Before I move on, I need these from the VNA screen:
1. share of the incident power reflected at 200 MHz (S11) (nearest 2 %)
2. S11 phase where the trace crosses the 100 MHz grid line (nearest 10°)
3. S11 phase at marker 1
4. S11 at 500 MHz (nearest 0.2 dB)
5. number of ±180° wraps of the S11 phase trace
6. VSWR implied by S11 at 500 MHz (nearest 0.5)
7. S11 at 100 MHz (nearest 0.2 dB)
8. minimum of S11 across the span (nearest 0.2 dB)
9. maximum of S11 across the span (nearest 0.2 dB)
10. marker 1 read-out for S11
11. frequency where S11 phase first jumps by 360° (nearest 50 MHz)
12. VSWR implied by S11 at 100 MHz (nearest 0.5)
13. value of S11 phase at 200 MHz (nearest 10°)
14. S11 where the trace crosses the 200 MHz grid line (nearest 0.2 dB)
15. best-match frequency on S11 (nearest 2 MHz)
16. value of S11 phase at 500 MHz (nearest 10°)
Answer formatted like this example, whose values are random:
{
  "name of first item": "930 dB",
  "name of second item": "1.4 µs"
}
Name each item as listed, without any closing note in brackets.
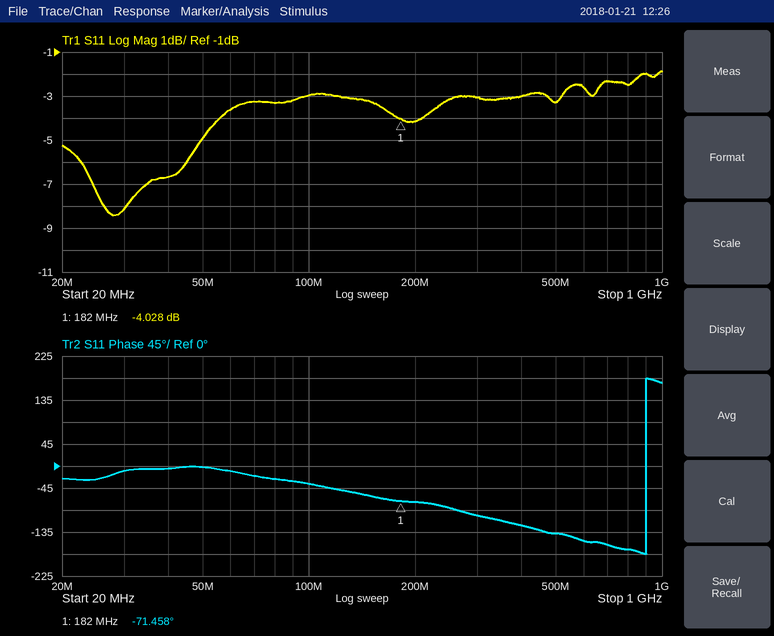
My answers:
{
  "share of the incident power reflected at 200 MHz (S11)": "38 %",
  "S11 phase where the trace crosses the 100 MHz grid line": "-40°",
  "S11 phase at marker 1": "-71.458°",
  "S11 at 500 MHz": "-3.2 dB",
  "number of ±180° wraps of the S11 phase trace": "1",
  "VSWR implied by S11 at 500 MHz": "5.5",
  "S11 at 100 MHz": "-3.0 dB",
  "minimum of S11 across the span": "-8.4 dB",
  "maximum of S11 across the span": "-1.8 dB",
  "marker 1 read-out for S11": "-4.028 dB",
  "frequency where S11 phase first jumps by 360°": "900 MHz",
  "VSWR implied by S11 at 100 MHz": "6.0",
  "value of S11 phase at 200 MHz": "-70°",
  "S11 where the trace crosses the 200 MHz grid line": "-4.2 dB",
  "best-match frequency on S11": "28 MHz",
  "value of S11 phase at 500 MHz": "-140°"
}
